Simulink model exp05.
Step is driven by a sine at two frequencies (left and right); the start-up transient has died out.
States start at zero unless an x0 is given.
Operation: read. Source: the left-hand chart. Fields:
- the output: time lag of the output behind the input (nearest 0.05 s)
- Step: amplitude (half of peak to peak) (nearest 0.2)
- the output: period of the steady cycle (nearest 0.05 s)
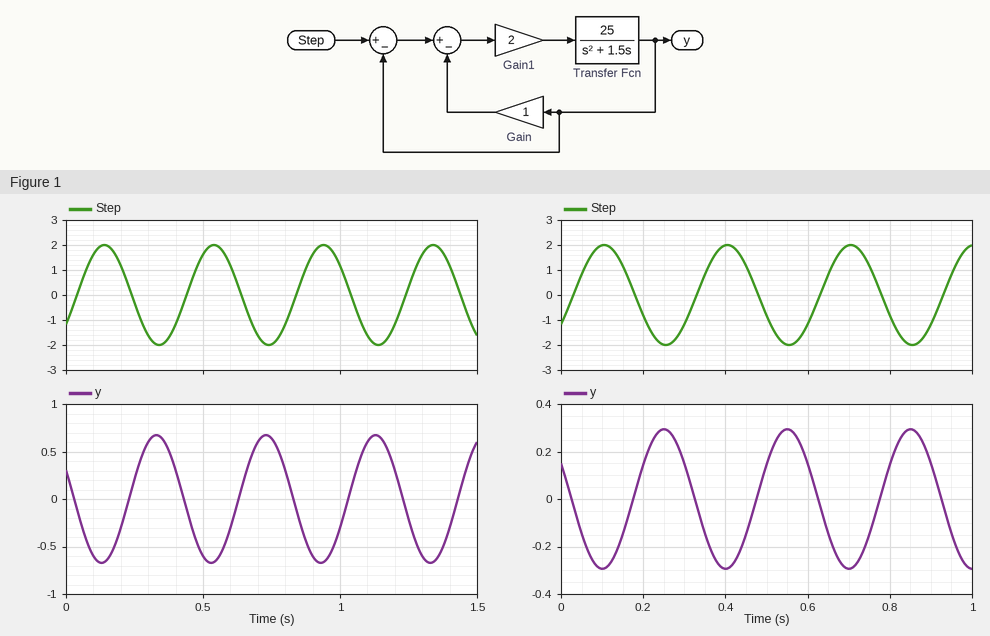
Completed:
0.20 s
2.0
0.40 s
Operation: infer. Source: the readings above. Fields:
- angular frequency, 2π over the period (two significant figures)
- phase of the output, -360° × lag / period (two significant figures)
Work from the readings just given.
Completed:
16 rad/s
-180°
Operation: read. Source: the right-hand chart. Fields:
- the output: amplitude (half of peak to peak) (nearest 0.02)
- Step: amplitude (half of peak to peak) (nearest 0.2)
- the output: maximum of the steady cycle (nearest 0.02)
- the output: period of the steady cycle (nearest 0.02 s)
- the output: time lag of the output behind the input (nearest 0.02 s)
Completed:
0.30
2.0
0.30
0.30 s
0.14 s
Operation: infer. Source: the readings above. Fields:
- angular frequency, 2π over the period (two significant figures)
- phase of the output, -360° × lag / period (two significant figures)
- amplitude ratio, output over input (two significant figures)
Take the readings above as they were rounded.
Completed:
21 rad/s
-170°
0.15
